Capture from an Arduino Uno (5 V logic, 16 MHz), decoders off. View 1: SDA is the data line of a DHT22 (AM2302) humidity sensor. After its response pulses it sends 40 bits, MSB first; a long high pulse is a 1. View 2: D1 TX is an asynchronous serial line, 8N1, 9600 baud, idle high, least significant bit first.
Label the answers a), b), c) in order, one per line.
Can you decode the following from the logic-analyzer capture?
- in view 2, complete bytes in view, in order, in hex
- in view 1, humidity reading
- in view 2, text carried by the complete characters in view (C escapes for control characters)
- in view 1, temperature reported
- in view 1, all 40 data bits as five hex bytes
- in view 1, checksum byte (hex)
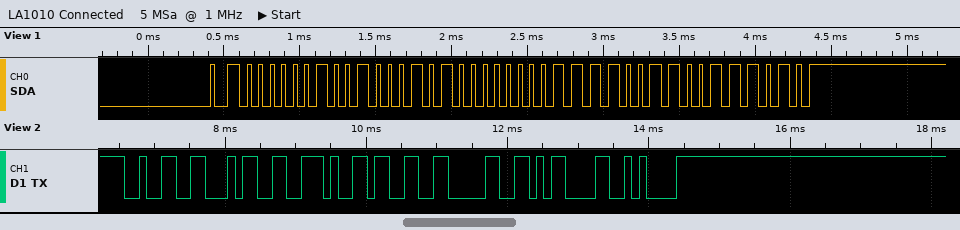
a) 0x32 0x34 0x2E 0x33 0x30 0x0D 0x0A
b) 58.1 %
c) "24.30\r\n"
d) 24.3 °C
e) 02 45 00 F3 3A
f) 0x3A
